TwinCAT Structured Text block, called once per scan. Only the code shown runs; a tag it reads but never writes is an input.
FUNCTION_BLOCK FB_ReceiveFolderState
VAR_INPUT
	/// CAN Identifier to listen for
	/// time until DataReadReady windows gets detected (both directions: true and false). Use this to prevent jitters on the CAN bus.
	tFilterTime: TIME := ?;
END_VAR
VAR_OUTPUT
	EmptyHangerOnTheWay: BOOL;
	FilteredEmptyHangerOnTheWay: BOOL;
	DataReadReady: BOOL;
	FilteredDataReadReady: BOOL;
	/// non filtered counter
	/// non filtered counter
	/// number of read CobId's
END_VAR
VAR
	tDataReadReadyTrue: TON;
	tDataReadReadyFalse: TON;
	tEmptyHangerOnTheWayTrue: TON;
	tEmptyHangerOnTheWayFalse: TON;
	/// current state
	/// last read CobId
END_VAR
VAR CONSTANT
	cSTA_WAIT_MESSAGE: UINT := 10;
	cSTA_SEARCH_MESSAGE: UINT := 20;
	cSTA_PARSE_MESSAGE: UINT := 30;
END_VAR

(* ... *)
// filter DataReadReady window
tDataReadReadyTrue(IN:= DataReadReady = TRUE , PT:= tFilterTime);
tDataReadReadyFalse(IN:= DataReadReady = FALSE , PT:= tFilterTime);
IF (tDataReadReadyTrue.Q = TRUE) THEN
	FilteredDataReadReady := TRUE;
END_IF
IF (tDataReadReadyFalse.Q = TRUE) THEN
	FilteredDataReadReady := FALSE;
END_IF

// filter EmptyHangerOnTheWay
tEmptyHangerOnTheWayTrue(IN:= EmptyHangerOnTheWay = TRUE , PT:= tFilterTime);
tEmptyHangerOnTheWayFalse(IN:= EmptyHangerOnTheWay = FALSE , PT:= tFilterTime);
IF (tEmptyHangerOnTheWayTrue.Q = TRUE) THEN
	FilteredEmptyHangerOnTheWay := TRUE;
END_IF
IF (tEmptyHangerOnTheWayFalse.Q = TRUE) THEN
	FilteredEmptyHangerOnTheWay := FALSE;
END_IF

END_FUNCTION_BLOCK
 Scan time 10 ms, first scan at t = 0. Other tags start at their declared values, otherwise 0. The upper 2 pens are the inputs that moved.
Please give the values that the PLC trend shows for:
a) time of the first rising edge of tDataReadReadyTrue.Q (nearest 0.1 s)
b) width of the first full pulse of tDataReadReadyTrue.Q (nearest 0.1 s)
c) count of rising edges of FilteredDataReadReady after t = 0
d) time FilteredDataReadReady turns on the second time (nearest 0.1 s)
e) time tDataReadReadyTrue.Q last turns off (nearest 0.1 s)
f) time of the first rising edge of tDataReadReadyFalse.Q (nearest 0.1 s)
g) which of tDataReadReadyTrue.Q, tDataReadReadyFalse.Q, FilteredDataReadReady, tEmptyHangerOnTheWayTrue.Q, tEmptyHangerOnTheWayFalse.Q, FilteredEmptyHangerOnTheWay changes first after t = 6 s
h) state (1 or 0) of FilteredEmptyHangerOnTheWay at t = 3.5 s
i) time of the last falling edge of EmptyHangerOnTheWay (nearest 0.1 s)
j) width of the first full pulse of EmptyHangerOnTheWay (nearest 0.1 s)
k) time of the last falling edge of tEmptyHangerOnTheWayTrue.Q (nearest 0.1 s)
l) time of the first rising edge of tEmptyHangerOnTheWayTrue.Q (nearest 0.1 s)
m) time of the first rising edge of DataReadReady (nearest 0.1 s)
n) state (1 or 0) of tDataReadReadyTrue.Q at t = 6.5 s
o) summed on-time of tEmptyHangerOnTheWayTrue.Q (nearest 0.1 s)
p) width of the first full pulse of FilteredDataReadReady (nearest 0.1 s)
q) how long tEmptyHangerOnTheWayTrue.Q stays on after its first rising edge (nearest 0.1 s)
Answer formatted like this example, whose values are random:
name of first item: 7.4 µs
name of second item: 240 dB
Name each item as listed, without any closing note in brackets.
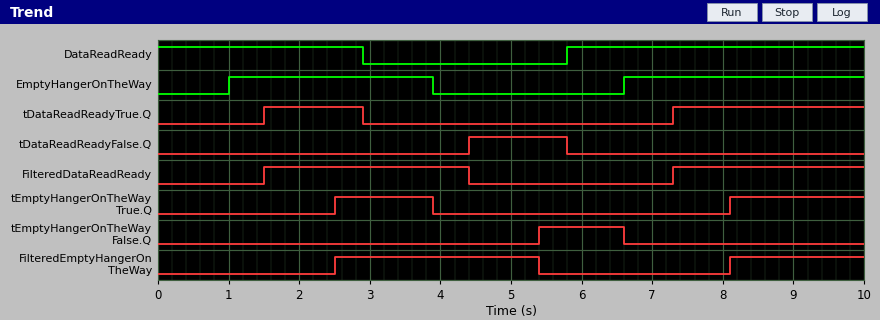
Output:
time of the first rising edge of tDataReadReadyTrue.Q: 1.5 s
width of the first full pulse of tDataReadReadyTrue.Q: 1.4 s
count of rising edges of FilteredDataReadReady after t = 0: 2
time FilteredDataReadReady turns on the second time: 7.3 s
time tDataReadReadyTrue.Q last turns off: 2.9 s
time of the first rising edge of tDataReadReadyFalse.Q: 4.4 s
which of tDataReadReadyTrue.Q, tDataReadReadyFalse.Q, FilteredDataReadReady, tEmptyHangerOnTheWayTrue.Q, tEmptyHangerOnTheWayFalse.Q, FilteredEmptyHangerOnTheWay changes first after t = 6 s: tEmptyHangerOnTheWayFalse.Q
state (1 or 0) of FilteredEmptyHangerOnTheWay at t = 3.5 s: 1
time of the last falling edge of EmptyHangerOnTheWay: 3.9 s
width of the first full pulse of EmptyHangerOnTheWay: 2.9 s
time of the last falling edge of tEmptyHangerOnTheWayTrue.Q: 3.9 s
time of the first rising edge of tEmptyHangerOnTheWayTrue.Q: 2.5 s
time of the first rising edge of DataReadReady: 5.8 s
state (1 or 0) of tDataReadReadyTrue.Q at t = 6.5 s: 0
summed on-time of tEmptyHangerOnTheWayTrue.Q: 3.3 s
width of the first full pulse of FilteredDataReadReady: 2.9 s
how long tEmptyHangerOnTheWayTrue.Q stays on after its first rising edge: 1.4 s
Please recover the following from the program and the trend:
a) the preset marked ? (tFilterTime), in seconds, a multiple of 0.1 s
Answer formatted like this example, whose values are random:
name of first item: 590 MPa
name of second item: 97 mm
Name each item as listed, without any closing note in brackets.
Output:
the preset marked ? (tFilterTime), in seconds, a multiple of 0.1 s: 1.5 s
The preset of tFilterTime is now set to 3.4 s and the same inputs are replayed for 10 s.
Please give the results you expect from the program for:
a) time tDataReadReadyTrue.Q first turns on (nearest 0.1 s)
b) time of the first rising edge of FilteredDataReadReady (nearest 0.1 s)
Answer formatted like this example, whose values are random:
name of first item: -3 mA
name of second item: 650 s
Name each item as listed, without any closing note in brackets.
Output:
time tDataReadReadyTrue.Q first turns on: 9.2 s
time of the first rising edge of FilteredDataReadReady: 9.2 s
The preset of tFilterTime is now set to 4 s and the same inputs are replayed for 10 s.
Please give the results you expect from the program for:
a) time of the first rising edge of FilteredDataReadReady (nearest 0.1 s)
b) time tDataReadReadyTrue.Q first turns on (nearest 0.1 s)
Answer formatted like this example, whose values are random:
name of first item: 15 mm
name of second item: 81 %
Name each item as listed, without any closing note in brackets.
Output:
time of the first rising edge of FilteredDataReadReady: 9.8 s
time tDataReadReadyTrue.Q first turns on: 9.8 s
